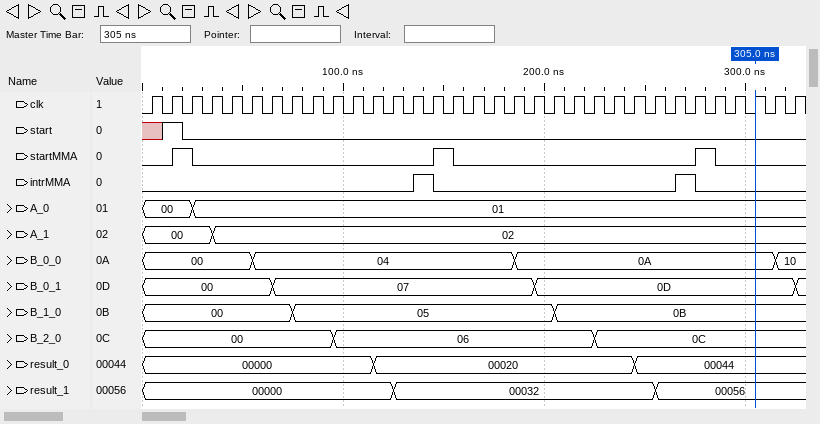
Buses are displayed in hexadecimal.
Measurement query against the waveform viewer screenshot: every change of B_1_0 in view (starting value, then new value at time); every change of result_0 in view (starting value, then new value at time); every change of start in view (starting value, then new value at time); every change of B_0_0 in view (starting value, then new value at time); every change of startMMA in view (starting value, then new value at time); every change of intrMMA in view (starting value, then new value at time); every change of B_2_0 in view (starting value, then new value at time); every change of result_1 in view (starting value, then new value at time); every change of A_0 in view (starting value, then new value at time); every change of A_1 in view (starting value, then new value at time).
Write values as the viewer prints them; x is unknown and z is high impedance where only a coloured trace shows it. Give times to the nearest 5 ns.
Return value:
00, 05 at 75 ns, 0B at 205 ns
00000, 00020 at 115 ns, 00044 at 245 ns
x, 1 at 10 ns, 0 at 20 ns
00, 04 at 55 ns, 0A at 185 ns, 10 at 315 ns
0, 1 at 15 ns, 0 at 25 ns, 1 at 145 ns, 0 at 155 ns, 1 at 275 ns, 0 at 285 ns
0, 1 at 135 ns, 0 at 145 ns, 1 at 265 ns, 0 at 275 ns
00, 06 at 95 ns, 0C at 225 ns
00000, 00032 at 125 ns, 00056 at 255 ns
00, 01 at 25 ns
00, 02 at 35 ns
